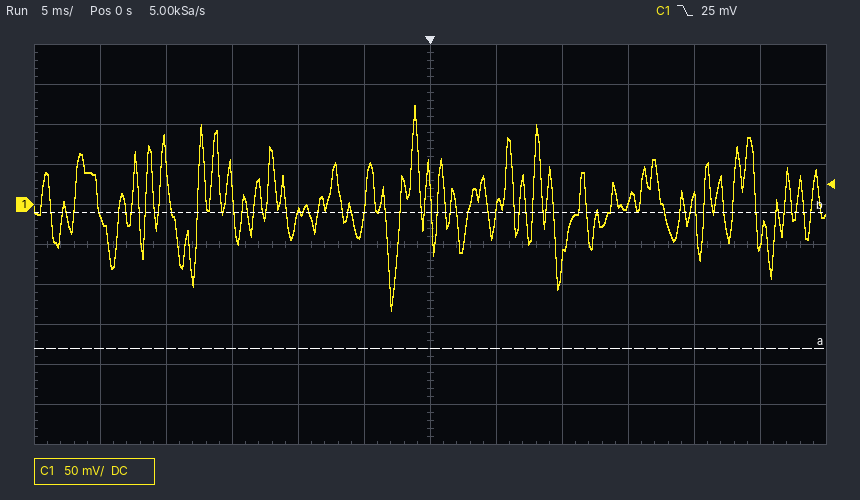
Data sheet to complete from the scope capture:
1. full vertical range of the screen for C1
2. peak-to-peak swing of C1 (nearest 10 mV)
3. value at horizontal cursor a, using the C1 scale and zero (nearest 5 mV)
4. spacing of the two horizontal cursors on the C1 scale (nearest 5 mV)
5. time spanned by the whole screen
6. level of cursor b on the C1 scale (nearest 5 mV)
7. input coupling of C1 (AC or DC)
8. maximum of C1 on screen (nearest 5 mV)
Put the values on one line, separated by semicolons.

500 mV; 260 mV; -180 mV; 170 mV; 60 ms; -10 mV; DC; 125 mV
